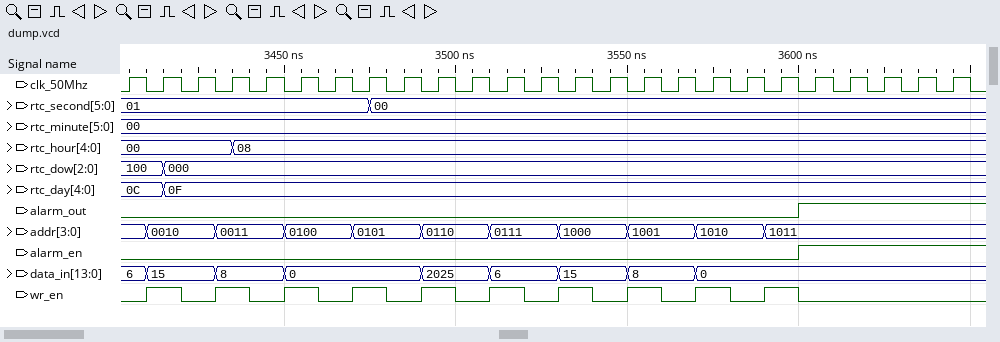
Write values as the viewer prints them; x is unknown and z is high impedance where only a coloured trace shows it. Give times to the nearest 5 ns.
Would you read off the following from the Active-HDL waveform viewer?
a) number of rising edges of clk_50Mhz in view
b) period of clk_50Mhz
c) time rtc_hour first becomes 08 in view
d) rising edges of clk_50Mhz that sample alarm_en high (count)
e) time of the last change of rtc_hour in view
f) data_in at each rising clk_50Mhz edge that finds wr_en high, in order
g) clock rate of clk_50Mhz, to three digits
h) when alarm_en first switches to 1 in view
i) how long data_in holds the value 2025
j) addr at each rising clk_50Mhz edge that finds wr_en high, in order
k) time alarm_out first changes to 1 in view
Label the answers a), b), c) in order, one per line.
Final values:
a) 25
b) 10 ns
c) 3435 ns
d) 5
e) 3435 ns
f) 15, 8, 0, 0, 2025, 6, 15, 8, 0, 0
g) 100 MHz
h) 3600 ns
i) 20 ns
j) 0010, 0011, 0100, 0101, 0110, 0111, 1000, 1001, 1010, 1011
k) 3600 ns
